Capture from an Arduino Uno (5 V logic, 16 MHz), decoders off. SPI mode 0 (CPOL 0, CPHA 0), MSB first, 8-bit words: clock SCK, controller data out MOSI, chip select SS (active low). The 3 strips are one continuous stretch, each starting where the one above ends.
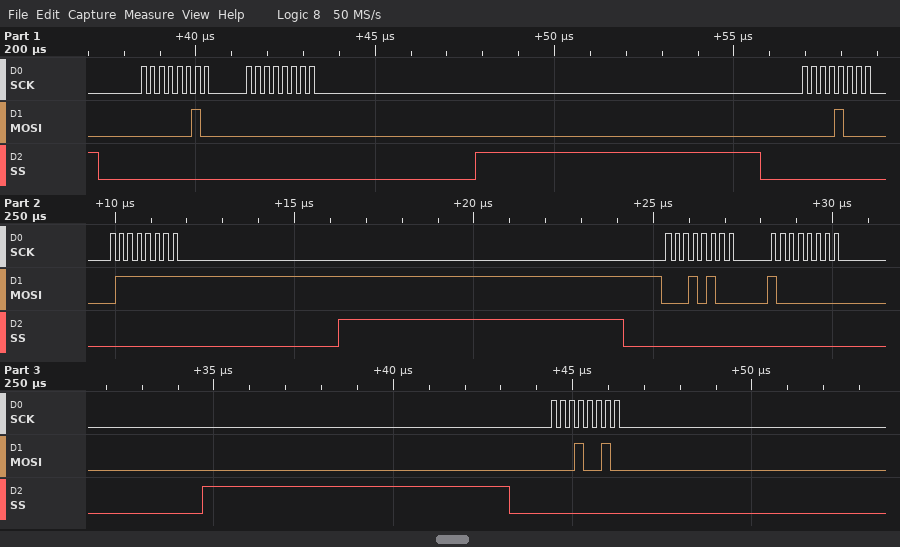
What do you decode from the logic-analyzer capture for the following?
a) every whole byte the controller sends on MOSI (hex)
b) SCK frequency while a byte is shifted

02 00 08 7F 14 80 12
4 MHz
